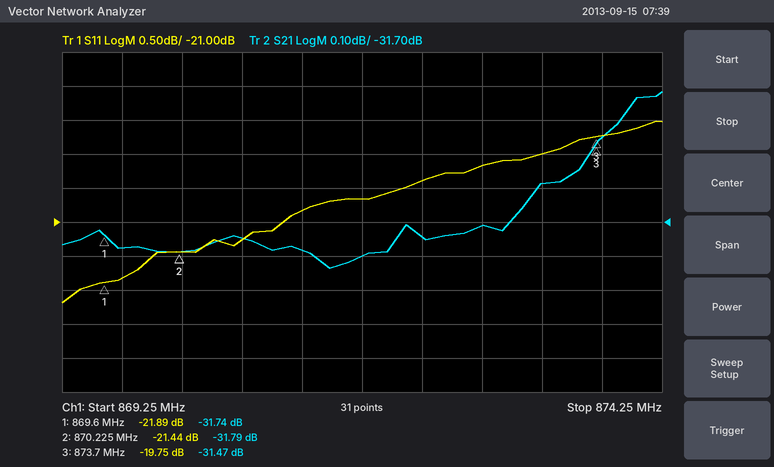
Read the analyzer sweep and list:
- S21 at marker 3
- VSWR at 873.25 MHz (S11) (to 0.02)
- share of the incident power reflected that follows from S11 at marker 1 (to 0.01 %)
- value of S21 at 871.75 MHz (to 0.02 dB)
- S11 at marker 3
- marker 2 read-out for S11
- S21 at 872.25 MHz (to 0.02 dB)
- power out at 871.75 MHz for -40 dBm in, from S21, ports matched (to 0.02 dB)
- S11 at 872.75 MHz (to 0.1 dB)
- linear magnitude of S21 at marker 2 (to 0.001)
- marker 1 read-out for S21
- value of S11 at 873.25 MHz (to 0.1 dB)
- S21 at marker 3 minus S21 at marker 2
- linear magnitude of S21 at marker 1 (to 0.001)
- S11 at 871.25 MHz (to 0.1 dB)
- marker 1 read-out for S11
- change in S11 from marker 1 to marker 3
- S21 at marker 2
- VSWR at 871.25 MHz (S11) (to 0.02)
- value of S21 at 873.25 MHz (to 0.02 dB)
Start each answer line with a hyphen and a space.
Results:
- -31.47 dB
- 1.22
- 0.65 %
- -31.80 dB
- -19.75 dB
- -21.44 dB
- -31.74 dB
- -71.80 dBm
- -20.2 dB
- 0.026
- -31.74 dB
- -20.0 dB
- 0.32 dB
- 0.026
- -20.8 dB
- -21.89 dB
- 2.14 dB
- -31.79 dB
- 1.20
- -31.58 dB
